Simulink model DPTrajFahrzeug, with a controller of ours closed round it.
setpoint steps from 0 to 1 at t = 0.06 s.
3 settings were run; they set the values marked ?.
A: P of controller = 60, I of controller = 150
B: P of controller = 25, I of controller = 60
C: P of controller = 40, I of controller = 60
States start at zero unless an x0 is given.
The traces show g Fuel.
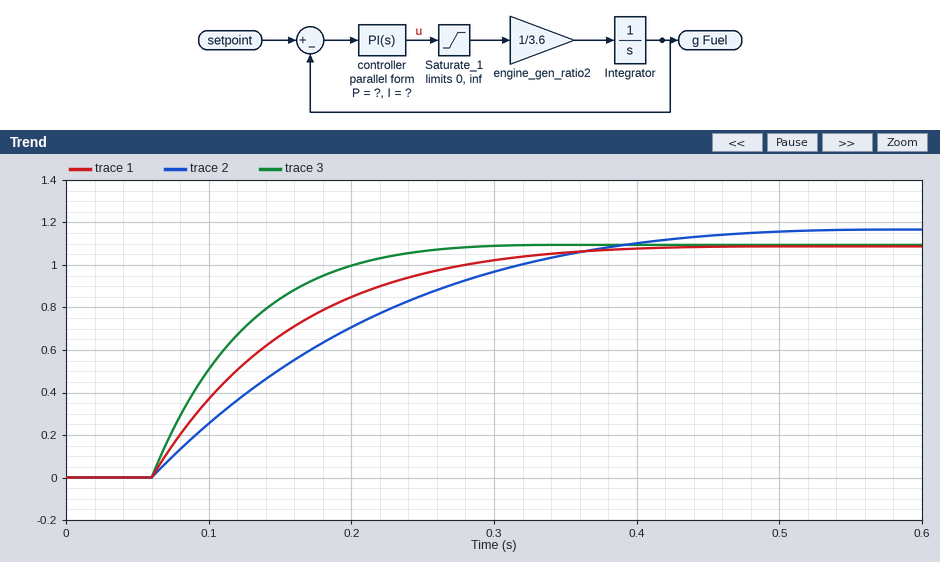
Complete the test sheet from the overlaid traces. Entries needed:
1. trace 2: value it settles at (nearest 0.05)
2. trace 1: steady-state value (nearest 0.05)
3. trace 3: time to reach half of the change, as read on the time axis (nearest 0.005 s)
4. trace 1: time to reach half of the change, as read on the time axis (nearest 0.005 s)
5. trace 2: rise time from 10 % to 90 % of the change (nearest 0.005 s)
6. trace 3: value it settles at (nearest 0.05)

1.15
1.10
0.105 s
0.125 s
0.275 s
1.10
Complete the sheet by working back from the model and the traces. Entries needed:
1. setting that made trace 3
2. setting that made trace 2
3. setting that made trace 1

A
B
C
